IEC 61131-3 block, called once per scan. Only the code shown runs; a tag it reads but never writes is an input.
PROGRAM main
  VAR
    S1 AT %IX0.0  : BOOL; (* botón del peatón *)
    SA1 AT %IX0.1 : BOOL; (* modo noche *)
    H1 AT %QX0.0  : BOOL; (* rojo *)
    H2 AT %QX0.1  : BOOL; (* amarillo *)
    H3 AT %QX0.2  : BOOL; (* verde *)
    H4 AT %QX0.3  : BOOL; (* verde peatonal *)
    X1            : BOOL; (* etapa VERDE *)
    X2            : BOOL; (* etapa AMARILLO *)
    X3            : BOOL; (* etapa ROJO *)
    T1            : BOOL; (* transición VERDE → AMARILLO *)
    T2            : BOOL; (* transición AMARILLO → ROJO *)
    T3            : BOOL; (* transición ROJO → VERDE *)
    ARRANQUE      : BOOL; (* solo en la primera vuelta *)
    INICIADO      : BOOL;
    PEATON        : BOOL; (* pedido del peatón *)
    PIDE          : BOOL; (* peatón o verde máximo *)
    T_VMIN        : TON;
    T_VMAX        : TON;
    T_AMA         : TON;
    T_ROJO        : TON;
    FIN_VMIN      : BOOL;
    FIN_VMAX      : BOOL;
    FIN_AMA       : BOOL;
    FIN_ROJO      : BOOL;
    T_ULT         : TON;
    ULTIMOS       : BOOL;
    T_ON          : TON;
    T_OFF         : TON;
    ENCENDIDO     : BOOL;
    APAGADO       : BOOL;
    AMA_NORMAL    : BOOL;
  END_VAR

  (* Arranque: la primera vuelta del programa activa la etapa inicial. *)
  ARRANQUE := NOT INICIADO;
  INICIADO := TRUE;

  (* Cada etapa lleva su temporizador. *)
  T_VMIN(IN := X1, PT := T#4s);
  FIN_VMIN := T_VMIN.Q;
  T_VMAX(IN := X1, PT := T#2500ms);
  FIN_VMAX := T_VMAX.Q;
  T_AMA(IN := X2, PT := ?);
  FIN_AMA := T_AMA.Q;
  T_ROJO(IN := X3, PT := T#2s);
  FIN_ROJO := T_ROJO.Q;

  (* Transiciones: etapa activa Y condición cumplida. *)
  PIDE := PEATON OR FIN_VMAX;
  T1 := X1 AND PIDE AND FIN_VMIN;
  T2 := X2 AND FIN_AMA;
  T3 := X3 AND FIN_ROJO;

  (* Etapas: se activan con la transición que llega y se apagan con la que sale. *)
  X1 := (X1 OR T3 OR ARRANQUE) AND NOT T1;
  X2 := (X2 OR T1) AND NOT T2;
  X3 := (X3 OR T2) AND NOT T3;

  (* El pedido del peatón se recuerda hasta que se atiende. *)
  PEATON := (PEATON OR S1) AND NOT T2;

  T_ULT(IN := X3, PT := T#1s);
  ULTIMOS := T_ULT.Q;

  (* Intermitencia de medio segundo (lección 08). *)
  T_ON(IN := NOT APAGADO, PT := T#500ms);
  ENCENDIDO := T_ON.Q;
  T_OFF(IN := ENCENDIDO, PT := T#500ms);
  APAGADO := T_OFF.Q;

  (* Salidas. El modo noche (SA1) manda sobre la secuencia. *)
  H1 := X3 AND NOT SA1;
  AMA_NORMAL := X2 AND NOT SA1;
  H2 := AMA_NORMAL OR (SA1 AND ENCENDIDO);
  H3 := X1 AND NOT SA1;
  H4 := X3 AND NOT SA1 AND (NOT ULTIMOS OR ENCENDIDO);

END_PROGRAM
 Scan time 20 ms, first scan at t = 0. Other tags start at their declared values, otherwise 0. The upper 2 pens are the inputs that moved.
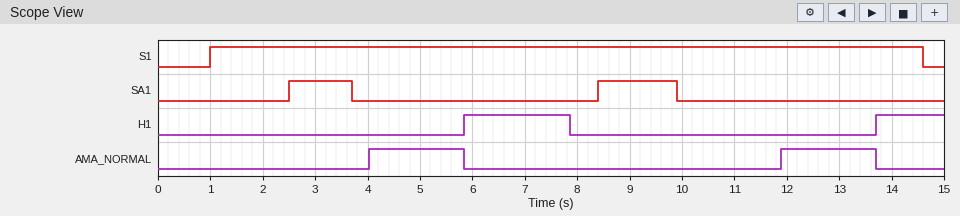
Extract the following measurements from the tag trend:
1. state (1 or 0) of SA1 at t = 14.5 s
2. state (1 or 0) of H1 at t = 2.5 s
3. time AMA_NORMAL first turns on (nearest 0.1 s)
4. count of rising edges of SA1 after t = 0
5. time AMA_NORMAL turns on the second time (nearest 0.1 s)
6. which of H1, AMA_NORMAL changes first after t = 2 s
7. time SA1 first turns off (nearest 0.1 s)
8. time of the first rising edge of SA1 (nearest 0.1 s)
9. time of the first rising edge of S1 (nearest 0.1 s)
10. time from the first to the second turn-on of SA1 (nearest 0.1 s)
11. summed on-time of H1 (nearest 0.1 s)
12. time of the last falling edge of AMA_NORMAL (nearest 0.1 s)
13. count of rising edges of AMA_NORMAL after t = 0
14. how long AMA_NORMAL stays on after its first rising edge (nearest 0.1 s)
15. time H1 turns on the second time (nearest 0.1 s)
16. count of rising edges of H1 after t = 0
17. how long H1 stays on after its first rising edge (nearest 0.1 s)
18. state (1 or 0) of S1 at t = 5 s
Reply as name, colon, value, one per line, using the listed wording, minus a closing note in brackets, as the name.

state (1 or 0) of SA1 at t = 14.5 s: 0
state (1 or 0) of H1 at t = 2.5 s: 0
time AMA_NORMAL first turns on: 4.0 s
count of rising edges of SA1 after t = 0: 2
time AMA_NORMAL turns on the second time: 11.9 s
which of H1, AMA_NORMAL changes first after t = 2 s: AMA_NORMAL
time SA1 first turns off: 3.7 s
time of the first rising edge of SA1: 2.5 s
time of the first rising edge of S1: 1.0 s
time from the first to the second turn-on of SA1: 5.9 s
summed on-time of H1: 3.3 s
time of the last falling edge of AMA_NORMAL: 13.7 s
count of rising edges of AMA_NORMAL after t = 0: 2
how long AMA_NORMAL stays on after its first rising edge: 1.8 s
time H1 turns on the second time: 13.7 s
count of rising edges of H1 after t = 0: 2
how long H1 stays on after its first rising edge: 2.0 s
state (1 or 0) of S1 at t = 5 s: 1
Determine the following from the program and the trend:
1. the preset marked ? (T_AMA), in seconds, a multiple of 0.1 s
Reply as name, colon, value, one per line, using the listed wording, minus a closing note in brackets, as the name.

the preset marked ? (T_AMA), in seconds, a multiple of 0.1 s: 1.8 s
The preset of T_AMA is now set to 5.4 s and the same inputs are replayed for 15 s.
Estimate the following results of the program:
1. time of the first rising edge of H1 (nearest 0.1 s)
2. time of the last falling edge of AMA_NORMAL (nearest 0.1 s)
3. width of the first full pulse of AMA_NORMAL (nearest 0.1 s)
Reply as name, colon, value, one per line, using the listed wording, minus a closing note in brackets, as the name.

time of the first rising edge of H1: 9.9 s
time of the last falling edge of AMA_NORMAL: 8.4 s
width of the first full pulse of AMA_NORMAL: 4.4 s
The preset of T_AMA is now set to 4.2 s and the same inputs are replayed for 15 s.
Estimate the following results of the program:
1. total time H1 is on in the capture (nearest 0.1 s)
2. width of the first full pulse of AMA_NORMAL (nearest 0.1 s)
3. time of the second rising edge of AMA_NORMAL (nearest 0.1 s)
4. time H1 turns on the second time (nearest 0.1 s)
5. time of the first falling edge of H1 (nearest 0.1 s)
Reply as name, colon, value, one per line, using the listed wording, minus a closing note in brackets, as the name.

total time H1 is on in the capture: 0.5 s
width of the first full pulse of AMA_NORMAL: 4.2 s
time of the second rising edge of AMA_NORMAL: 14.3 s
time H1 turns on the second time: 9.9 s
time of the first falling edge of H1: 8.4 s
